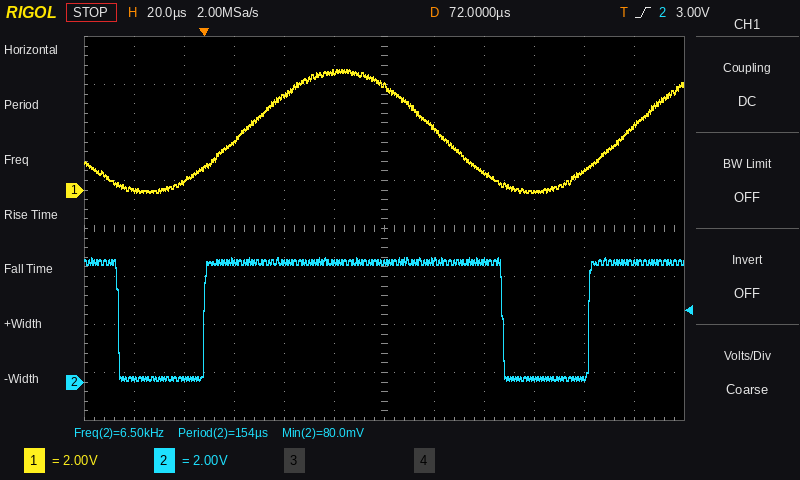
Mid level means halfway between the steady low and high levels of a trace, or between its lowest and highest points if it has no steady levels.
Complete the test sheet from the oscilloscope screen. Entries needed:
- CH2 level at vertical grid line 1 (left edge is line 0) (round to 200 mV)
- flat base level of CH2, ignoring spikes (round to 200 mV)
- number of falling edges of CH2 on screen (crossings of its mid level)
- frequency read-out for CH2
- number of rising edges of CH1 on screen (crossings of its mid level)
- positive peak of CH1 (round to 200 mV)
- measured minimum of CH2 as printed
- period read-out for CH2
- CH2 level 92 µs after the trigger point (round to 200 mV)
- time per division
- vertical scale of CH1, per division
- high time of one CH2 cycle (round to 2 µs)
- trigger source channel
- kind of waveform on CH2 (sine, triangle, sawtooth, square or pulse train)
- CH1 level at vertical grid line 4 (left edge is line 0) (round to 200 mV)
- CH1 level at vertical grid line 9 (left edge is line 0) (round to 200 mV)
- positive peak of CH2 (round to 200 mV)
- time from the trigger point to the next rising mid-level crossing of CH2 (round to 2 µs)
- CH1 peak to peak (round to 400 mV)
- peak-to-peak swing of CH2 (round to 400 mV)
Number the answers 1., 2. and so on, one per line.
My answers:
1. 200 mV
2. 200 mV
3. 2
4. 6.50 kHz
5. 2
6. 5.0 V
7. 80.0 mV
8. 154 µs
9. 5.0 V
10. 20 µs
11. 2 V
12. 120 µs
13. CH2
14. pulse train
15. 4.0 V
16. 0.0 V
17. 5.2 V
18. 154 µs
19. 5.2 V
20. 5.2 V
